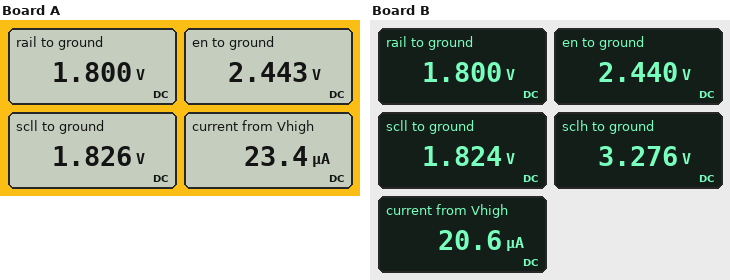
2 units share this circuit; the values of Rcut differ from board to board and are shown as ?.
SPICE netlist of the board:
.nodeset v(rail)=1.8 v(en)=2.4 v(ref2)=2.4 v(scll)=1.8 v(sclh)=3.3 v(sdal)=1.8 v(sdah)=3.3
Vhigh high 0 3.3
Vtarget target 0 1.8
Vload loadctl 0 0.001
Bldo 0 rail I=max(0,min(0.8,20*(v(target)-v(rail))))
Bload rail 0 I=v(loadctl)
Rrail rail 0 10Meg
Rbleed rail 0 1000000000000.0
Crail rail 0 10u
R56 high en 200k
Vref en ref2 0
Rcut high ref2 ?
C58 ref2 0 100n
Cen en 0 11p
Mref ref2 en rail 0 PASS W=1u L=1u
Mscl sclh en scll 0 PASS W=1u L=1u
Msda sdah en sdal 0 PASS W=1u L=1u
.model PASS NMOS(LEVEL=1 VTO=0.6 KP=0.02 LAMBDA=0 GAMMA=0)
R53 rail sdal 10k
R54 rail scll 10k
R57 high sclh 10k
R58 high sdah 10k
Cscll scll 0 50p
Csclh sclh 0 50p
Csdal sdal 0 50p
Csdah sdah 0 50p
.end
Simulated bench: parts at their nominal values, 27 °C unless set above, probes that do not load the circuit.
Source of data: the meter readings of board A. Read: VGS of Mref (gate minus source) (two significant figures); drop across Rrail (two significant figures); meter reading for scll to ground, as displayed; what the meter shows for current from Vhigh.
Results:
640 mV
1.8 V
1.826 V
23.4 µA
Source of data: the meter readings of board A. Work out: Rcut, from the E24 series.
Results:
62 kΩ
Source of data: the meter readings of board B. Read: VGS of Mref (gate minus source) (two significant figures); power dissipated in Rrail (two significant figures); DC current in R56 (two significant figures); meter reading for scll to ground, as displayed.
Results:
640 mV
320 nW
4.3 µA
1.824 V
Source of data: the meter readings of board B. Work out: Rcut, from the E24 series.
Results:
75 kΩ
